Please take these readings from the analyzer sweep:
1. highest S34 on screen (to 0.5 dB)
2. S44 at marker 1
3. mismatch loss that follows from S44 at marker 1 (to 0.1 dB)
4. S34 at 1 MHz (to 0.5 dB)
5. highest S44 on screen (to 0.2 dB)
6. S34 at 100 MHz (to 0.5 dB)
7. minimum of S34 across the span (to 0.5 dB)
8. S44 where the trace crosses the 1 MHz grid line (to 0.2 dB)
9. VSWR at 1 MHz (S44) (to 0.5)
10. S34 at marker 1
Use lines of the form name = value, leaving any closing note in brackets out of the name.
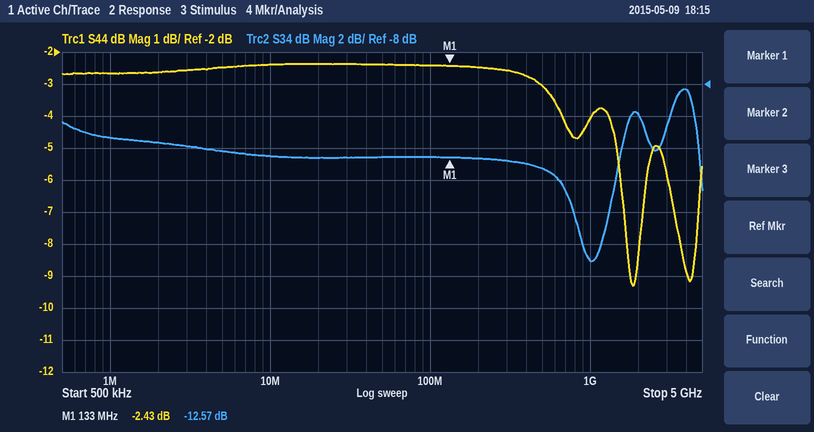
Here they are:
highest S34 on screen = -8.5 dB
S44 at marker 1 = -2.43 dB
mismatch loss that follows from S44 at marker 1 = 3.7 dB
S34 at 1 MHz = -11.5 dB
highest S44 on screen = -2.4 dB
S34 at 100 MHz = -12.5 dB
minimum of S34 across the span = -19.0 dB
S44 where the trace crosses the 1 MHz grid line = -2.6 dB
VSWR at 1 MHz (S44) = 6.5
S34 at marker 1 = -12.57 dB
